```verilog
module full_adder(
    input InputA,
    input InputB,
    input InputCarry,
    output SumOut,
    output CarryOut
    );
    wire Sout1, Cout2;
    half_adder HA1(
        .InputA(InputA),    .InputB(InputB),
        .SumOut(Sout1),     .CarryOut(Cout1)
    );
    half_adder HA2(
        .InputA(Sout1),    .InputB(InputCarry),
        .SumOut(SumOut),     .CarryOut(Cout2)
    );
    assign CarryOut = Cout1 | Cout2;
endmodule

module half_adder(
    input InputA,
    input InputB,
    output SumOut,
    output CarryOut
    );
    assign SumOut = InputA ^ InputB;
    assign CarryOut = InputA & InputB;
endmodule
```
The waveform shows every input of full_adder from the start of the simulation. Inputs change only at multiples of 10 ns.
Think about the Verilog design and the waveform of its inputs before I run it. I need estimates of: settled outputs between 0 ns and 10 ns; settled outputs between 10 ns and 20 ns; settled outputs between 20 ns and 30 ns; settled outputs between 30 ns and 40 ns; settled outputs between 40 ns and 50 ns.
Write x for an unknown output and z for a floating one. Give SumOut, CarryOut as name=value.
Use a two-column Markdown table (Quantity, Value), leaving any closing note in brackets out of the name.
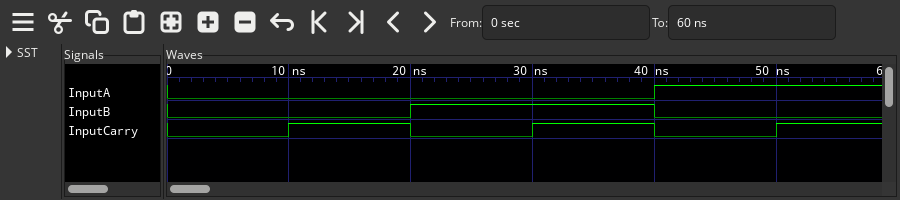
| Quantity | Value |
|---|---|
| settled outputs between 0 ns and 10 ns | SumOut=0, CarryOut=0 |
| settled outputs between 10 ns and 20 ns | SumOut=1, CarryOut=0 |
| settled outputs between 20 ns and 30 ns | SumOut=1, CarryOut=0 |
| settled outputs between 30 ns and 40 ns | SumOut=0, CarryOut=1 |
| settled outputs between 40 ns and 50 ns | SumOut=1, CarryOut=0 |
